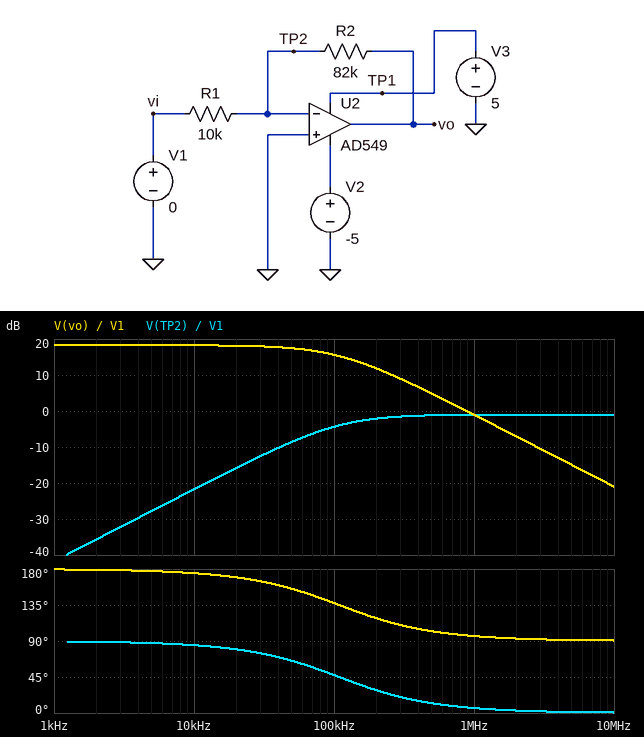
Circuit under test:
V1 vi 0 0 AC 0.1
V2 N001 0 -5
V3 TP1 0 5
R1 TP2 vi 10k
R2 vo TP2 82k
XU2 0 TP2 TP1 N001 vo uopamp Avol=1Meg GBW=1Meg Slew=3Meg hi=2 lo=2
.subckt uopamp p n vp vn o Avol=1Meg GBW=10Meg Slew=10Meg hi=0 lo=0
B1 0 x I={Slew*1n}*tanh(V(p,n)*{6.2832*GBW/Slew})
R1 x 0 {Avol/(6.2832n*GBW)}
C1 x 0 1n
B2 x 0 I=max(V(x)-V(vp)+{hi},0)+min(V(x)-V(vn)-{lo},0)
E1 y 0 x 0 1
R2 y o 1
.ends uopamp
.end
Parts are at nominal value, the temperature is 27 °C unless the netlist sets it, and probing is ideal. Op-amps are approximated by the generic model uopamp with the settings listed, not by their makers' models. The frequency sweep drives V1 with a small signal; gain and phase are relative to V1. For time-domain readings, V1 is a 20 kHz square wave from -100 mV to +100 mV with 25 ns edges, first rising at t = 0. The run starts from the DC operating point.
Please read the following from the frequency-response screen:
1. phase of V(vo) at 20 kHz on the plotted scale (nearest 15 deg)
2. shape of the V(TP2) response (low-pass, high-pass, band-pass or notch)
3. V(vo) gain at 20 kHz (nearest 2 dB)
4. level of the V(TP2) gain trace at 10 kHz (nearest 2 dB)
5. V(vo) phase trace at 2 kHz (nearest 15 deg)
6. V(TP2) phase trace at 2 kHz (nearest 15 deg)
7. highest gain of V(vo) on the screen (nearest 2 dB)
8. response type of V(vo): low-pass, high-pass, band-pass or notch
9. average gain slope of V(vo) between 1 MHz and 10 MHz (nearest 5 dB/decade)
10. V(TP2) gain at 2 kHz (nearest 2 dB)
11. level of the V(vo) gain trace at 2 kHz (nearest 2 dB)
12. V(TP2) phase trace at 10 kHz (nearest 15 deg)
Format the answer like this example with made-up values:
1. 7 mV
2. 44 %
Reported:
1. 165 deg
2. high-pass
3. 18 dB
4. -22 dB
5. 180 deg
6. 90 deg
7. 18 dB
8. low-pass
9. -20 dB/decade
10. -36 dB
11. 18 dB
12. 90 deg
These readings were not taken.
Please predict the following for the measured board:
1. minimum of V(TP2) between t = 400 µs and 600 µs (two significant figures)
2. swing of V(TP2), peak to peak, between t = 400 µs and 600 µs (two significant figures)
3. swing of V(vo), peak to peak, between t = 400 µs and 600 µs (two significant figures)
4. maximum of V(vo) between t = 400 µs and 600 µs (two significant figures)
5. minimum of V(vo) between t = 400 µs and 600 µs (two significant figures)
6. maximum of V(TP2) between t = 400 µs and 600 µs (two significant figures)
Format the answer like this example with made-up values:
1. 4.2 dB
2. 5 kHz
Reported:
1. -180 mV
2. 350 mV
3. 1.6 V
4. 820 mV
5. -820 mV
6. 180 mV
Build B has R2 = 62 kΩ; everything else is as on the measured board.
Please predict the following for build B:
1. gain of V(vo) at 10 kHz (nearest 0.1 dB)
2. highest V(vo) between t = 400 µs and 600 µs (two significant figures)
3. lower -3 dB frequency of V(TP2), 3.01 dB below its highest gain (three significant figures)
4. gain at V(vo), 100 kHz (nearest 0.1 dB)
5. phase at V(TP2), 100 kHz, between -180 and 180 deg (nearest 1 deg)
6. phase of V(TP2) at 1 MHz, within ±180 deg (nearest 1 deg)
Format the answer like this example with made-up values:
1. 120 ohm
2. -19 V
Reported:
1. 15.8 dB
2. 620 mV
3. 139 kHz
4. 14.0 dB
5. 54 deg
6. 8 deg
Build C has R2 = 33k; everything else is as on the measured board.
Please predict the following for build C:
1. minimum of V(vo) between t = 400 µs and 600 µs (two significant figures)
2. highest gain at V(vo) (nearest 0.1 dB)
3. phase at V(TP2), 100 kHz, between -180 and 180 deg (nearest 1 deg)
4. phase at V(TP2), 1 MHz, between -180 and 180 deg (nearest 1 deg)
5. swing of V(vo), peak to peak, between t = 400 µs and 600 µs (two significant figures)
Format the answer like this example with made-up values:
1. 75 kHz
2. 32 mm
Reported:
1. -330 mV
2. 10.4 dB
3. 67 deg
4. 13 deg
5. 660 mV
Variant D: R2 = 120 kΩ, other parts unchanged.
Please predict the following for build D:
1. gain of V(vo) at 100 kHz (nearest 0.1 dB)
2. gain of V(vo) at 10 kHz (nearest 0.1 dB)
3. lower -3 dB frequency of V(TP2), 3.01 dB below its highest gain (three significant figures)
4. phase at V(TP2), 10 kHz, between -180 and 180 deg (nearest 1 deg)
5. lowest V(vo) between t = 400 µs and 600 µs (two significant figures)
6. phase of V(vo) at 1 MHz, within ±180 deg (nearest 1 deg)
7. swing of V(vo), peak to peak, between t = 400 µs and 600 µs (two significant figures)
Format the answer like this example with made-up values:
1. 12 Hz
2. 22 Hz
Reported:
1. 17.3 dB
2. 21.5 dB
3. 76.9 kHz
4. 83 deg
5. -1.2 V
6. 94 deg
7. 2.4 V
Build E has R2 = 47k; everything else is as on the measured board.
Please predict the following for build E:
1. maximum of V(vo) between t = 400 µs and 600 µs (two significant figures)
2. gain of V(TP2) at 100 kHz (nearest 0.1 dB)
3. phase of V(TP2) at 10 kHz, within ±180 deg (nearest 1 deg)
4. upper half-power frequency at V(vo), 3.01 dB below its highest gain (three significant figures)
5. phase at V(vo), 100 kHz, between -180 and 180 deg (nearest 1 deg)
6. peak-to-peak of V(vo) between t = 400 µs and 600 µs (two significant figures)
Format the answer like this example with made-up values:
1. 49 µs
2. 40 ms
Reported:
1. 470 mV
2. -7.8 dB
3. 87 deg
4. 175 kHz
5. 150 deg
6. 940 mV
